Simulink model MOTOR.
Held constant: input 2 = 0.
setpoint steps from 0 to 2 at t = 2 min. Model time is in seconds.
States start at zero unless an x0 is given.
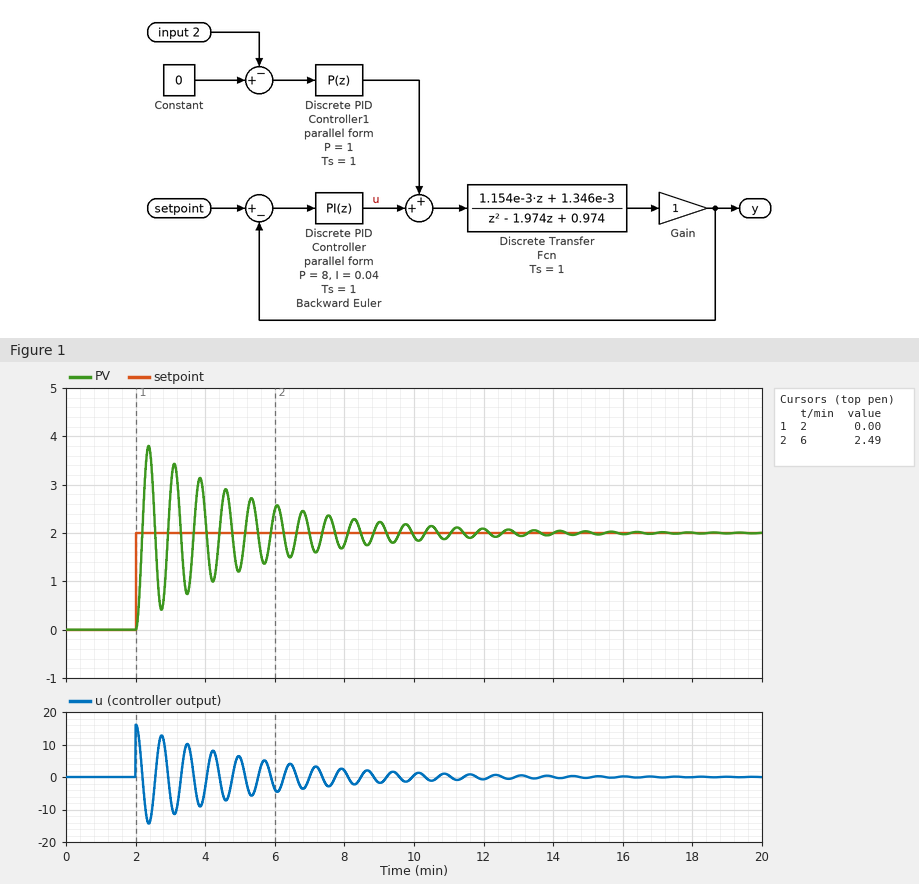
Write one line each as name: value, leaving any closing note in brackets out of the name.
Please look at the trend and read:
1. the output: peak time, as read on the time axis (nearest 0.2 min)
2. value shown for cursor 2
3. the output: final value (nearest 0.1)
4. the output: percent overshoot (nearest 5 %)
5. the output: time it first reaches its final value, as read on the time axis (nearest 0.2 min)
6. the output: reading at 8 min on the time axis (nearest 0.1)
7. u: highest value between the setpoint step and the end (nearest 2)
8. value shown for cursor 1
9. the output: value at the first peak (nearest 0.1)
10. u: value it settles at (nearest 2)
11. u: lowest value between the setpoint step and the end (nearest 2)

the output: peak time, as read on the time axis: 2.4 min
value shown for cursor 2: 2.49
the output: final value: 2.0
the output: percent overshoot: 90 %
the output: time it first reaches its final value, as read on the time axis: 2.2 min
the output: reading at 8 min on the time axis: 1.8
u: highest value between the setpoint step and the end: 16
value shown for cursor 1: 0.00
the output: value at the first peak: 3.8
u: value it settles at: 0
u: lowest value between the setpoint step and the end: -14
